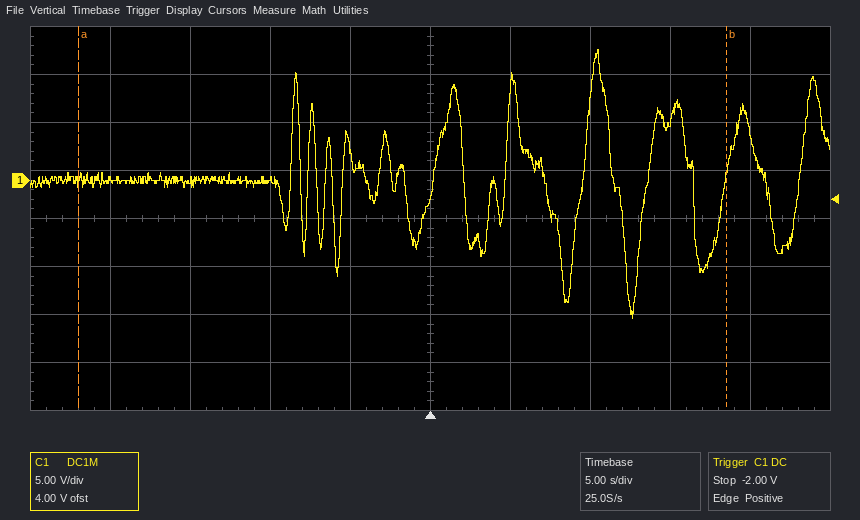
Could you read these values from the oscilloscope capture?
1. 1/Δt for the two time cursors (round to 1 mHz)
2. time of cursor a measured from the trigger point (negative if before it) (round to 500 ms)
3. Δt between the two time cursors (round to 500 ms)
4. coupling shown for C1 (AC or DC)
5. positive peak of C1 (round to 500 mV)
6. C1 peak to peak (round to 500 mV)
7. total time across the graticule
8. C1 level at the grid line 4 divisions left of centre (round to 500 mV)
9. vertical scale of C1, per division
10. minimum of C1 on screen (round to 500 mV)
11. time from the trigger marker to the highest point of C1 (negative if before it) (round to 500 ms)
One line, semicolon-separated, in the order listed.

25 mHz; -22.0 s; 40.5 s; DC; 13.5 V; 28.0 V; 50 s; 0.0 V; 5 V; -14.5 V; +10.5 s
